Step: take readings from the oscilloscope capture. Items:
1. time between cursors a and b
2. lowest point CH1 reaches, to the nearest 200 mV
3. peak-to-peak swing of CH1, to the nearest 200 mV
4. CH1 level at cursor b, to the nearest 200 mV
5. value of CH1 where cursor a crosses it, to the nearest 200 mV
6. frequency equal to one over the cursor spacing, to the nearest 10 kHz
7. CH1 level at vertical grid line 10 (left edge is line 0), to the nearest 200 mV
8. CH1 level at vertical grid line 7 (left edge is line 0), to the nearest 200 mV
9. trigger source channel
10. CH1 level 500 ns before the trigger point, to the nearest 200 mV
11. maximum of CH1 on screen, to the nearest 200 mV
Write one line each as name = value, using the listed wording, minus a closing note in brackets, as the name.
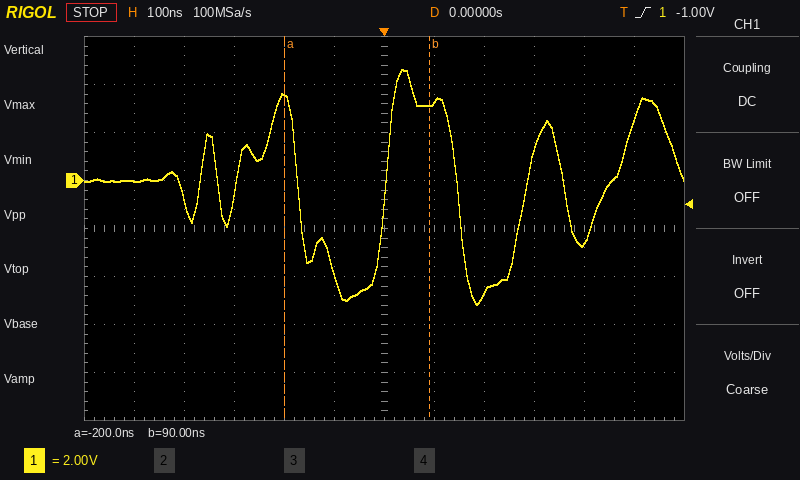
time between cursors a and b = 290 ns
lowest point CH1 reaches, to the nearest 200 mV = -5.2 V
peak-to-peak swing of CH1, to the nearest 200 mV = 9.8 V
CH1 level at cursor b, to the nearest 200 mV = 3.2 V
value of CH1 where cursor a crosses it, to the nearest 200 mV = 3.4 V
frequency equal to one over the cursor spacing, to the nearest 10 kHz = 3.45 MHz
CH1 level at vertical grid line 10 (left edge is line 0), to the nearest 200 mV = -2.6 V
CH1 level at vertical grid line 7 (left edge is line 0), to the nearest 200 mV = 3.2 V
trigger source channel = CH1
CH1 level 500 ns before the trigger point, to the nearest 200 mV = 0.0 V
maximum of CH1 on screen, to the nearest 200 mV = 4.6 V
